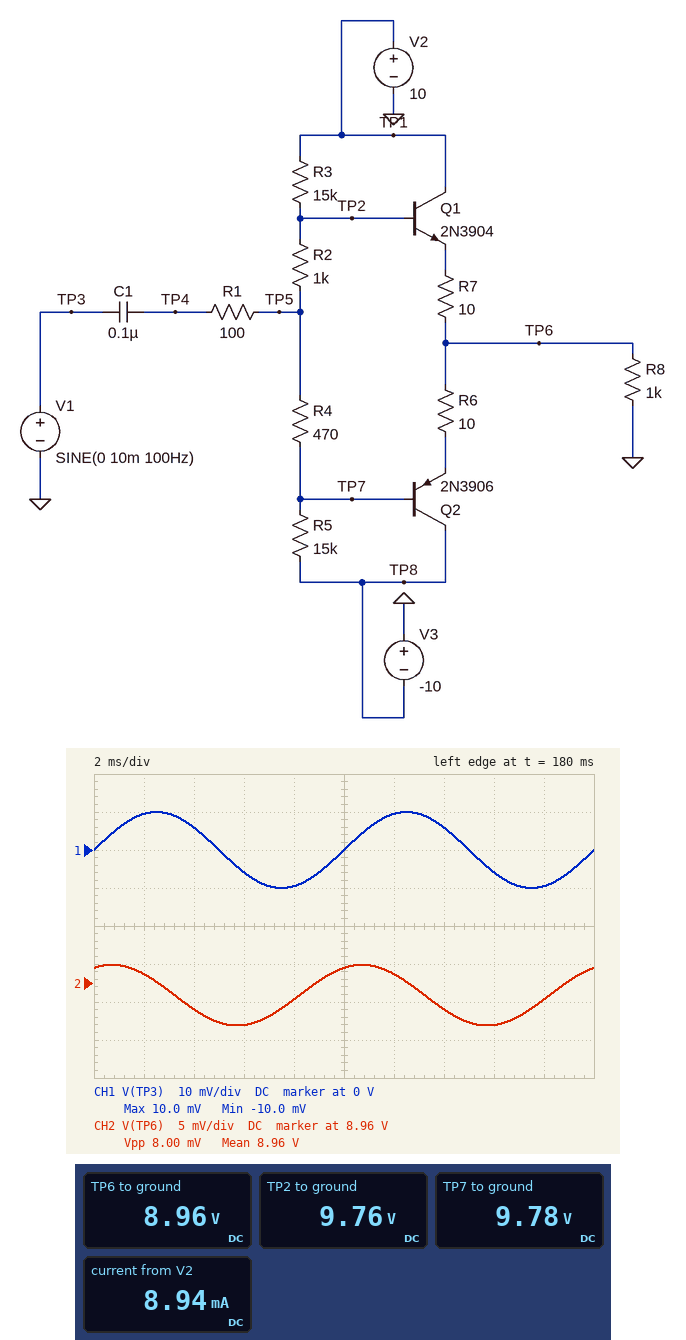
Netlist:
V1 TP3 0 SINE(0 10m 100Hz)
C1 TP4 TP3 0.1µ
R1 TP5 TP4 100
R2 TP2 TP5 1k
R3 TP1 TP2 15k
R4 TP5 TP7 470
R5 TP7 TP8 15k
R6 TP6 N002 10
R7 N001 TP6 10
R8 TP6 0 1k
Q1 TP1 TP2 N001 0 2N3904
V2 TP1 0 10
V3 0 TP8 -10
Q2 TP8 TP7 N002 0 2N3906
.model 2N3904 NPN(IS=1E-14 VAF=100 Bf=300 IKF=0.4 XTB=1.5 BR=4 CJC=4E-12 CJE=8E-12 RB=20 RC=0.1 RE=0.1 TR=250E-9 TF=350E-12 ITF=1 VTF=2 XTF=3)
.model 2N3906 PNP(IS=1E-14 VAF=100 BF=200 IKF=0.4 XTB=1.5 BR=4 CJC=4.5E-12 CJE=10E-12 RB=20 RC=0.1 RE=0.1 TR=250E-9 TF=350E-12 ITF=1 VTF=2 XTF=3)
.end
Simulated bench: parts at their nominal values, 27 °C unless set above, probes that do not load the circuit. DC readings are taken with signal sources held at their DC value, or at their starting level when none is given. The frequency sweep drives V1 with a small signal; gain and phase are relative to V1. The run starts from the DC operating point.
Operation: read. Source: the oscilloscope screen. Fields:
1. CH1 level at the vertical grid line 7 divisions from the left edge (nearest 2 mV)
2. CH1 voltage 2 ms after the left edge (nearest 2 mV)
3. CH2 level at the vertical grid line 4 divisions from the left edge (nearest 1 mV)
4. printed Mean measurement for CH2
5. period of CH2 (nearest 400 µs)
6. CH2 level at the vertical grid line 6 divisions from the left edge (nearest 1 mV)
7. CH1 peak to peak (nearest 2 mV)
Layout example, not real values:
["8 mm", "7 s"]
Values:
["6 mV", "10 mV", "8.958 V", "8.96 V", "10.0 ms", "8.961 V", "20 mV"]
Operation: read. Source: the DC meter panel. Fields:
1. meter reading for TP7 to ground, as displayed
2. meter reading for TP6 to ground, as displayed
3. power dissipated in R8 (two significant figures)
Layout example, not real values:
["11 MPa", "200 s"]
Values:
["9.78 V", "8.96 V", "80 mW"]
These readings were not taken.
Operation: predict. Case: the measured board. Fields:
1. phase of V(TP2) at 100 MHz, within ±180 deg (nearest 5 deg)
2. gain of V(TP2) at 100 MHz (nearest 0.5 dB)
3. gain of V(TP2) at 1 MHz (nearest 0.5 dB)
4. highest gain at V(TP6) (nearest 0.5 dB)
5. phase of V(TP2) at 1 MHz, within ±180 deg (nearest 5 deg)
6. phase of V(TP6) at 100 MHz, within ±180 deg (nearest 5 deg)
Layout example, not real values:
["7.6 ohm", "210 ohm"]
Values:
["-65 deg", "-11.0 dB", "-0.5 dB", "-1.0 dB", "0 deg", "-65 deg"]
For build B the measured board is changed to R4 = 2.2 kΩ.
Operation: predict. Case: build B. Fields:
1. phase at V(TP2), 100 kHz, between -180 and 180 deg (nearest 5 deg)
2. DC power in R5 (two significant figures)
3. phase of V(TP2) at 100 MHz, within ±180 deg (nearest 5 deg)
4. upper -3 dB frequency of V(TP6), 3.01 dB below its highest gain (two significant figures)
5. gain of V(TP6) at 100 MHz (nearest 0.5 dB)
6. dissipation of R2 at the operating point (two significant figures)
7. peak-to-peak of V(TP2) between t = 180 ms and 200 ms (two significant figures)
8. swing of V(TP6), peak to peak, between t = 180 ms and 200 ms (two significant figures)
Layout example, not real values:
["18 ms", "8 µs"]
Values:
["0 deg", "2.8 µW", "-70 deg", "38 MHz", "-10.0 dB", "190 nW", "8.4 mV", "8.3 mV"]
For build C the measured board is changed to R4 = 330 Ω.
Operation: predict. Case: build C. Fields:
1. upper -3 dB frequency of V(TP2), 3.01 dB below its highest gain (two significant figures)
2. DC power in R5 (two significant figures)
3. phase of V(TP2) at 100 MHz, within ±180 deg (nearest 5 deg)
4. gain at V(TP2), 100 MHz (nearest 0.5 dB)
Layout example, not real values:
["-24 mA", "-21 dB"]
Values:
["31 MHz", "3.2 µW", "-60 deg", "-11.5 dB"]
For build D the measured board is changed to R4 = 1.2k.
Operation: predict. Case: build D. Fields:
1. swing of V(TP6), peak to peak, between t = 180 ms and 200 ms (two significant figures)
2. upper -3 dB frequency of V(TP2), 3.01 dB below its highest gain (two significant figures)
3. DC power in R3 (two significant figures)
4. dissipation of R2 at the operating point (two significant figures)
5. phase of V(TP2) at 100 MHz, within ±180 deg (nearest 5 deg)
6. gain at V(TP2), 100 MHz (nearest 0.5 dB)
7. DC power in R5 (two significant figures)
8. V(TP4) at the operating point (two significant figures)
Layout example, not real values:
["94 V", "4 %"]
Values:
["8.1 mV", "36 MHz", "3.9 µW", "200 nW", "-70 deg", "-10.0 dB", "3.0 µW", "9.8 V"]
